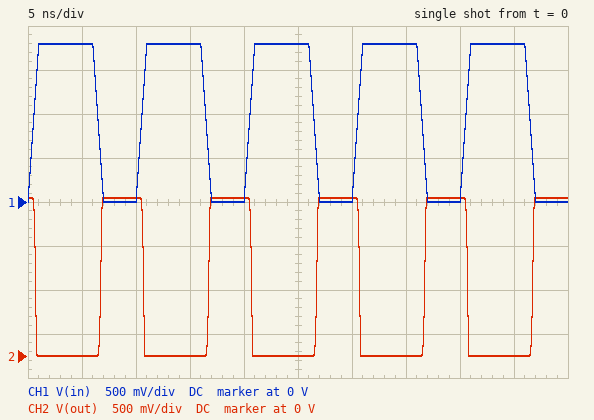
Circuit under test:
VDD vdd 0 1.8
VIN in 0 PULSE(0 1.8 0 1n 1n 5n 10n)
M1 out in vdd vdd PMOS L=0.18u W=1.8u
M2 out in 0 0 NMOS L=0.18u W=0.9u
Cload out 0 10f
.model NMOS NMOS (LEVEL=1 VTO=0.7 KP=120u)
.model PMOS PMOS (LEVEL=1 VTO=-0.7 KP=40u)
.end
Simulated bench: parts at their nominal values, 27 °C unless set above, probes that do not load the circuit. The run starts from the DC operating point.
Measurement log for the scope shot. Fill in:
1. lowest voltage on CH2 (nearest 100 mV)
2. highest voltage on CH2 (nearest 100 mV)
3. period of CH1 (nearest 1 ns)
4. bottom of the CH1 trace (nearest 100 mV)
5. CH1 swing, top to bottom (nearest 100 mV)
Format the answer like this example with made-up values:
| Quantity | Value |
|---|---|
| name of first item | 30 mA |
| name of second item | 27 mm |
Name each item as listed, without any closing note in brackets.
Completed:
| Quantity | Value |
|---|---|
| lowest voltage on CH2 | 0 V |
| highest voltage on CH2 | 1.8 V |
| period of CH1 | 10 ns |
| bottom of the CH1 trace | 0 V |
| CH1 swing, top to bottom | 1.8 V |
